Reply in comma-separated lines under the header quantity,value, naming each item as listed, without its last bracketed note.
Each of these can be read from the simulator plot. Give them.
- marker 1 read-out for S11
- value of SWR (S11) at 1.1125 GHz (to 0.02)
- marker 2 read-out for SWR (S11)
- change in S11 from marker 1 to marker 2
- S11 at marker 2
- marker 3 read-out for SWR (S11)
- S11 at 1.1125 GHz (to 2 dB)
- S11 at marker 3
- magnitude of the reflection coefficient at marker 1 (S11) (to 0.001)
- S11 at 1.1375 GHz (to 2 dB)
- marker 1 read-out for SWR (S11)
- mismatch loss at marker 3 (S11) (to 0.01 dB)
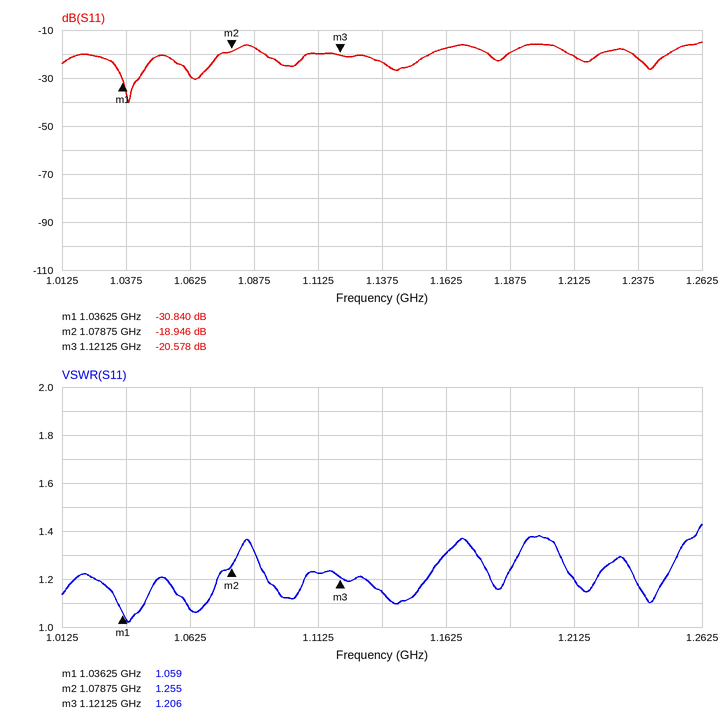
quantity,value
marker 1 read-out for S11,-30.840 dB
value of SWR (S11) at 1.1125 GHz,1.22
marker 2 read-out for SWR,1.255
change in S11 from marker 1 to marker 2,11.894 dB
S11 at marker 2,-18.946 dB
marker 3 read-out for SWR,1.206
S11 at 1.1125 GHz,-20 dB
S11 at marker 3,-20.578 dB
magnitude of the reflection coefficient at marker 1 (S11),0.029
S11 at 1.1375 GHz,-24 dB
marker 1 read-out for SWR,1.059
mismatch loss at marker 3 (S11),0.04 dB
